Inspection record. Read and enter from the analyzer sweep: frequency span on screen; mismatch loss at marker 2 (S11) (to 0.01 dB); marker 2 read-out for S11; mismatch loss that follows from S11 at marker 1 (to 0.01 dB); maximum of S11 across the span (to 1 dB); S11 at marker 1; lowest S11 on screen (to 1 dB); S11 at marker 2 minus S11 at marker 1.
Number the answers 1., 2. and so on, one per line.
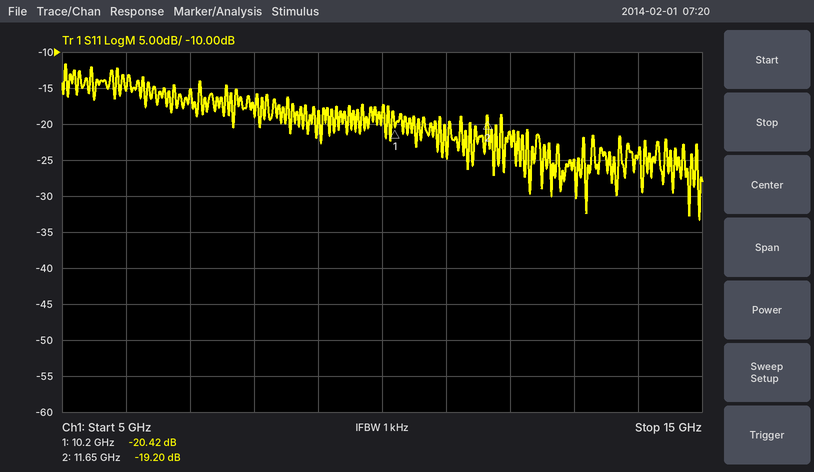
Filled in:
1. 10 GHz
2. 0.05 dB
3. -19.20 dB
4. 0.04 dB
5. -12 dB
6. -20.42 dB
7. -33 dB
8. 1.22 dB
